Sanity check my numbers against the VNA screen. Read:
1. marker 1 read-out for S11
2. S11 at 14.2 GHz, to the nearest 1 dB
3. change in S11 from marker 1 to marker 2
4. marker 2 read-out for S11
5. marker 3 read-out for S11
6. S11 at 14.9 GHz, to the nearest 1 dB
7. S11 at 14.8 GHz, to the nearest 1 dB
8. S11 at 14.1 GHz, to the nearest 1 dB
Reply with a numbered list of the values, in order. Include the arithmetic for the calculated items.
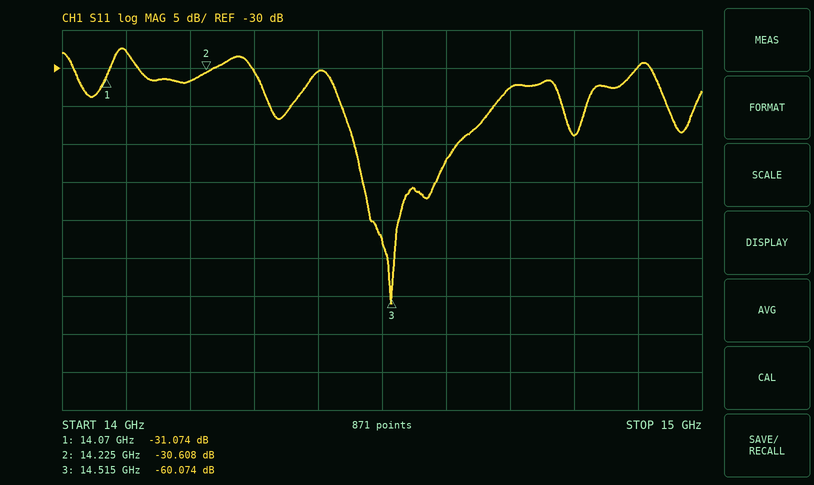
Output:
1. -31.074 dB
2. -32 dB
3. -30.608 − (-31.074) = 0.466 dB
4. -30.608 dB
5. -60.074 dB
6. -30 dB
7. -39 dB
8. -28 dB
